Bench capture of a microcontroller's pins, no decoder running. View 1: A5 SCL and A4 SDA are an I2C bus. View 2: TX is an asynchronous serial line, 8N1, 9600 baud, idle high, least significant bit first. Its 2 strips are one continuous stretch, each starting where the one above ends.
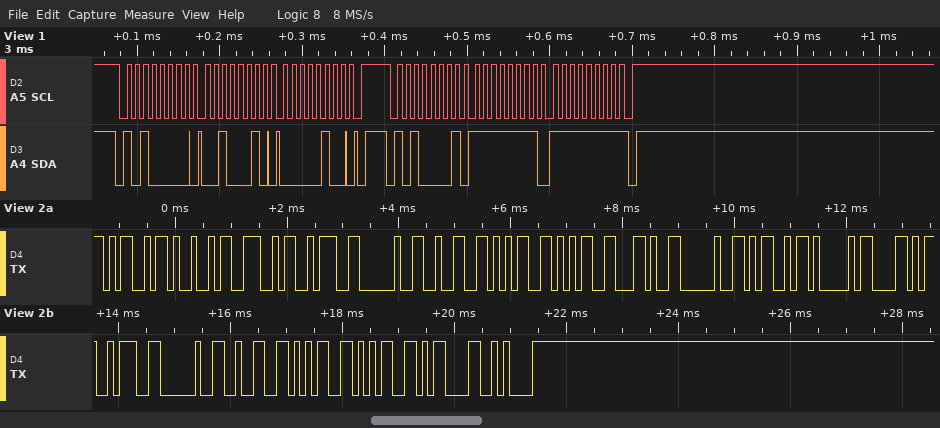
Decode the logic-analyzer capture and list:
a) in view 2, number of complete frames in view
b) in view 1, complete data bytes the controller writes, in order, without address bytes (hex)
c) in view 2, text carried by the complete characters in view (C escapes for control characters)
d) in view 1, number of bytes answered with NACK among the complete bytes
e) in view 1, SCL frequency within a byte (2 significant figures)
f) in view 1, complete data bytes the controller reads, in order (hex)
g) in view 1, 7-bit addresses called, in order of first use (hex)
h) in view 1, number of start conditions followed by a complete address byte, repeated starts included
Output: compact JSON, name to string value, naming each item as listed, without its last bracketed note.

{"in view 2, number of complete frames in view": "20", "in view 1, complete data bytes the controller writes, in order, without address bytes": "22 04", "in view 2, text carried by the complete characters in view": "\"MIN: 255, MAX: 255\\r\\n\"", "in view 1, number of bytes answered with NACK among the complete bytes": "1", "in view 1, SCL frequency within a byte": "100 kHz", "in view 1, complete data bytes the controller reads, in order": "FF FF", "in view 1, 7-bit addresses called, in order of first use": "0x50", "in view 1, number of start conditions followed by a complete address byte, repeated starts included": "2"}
